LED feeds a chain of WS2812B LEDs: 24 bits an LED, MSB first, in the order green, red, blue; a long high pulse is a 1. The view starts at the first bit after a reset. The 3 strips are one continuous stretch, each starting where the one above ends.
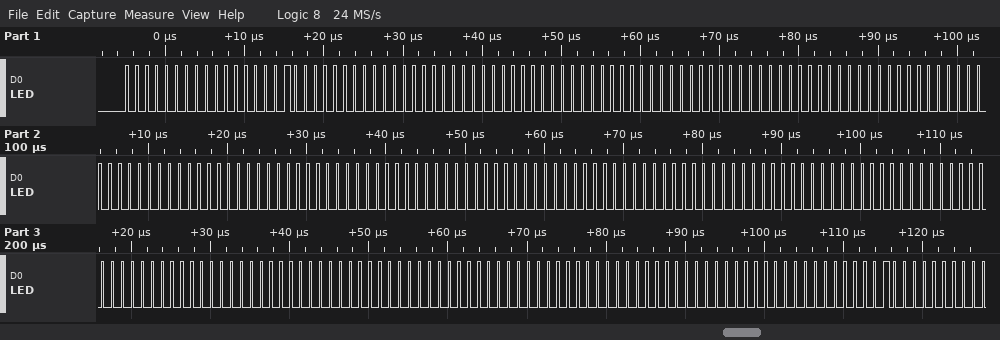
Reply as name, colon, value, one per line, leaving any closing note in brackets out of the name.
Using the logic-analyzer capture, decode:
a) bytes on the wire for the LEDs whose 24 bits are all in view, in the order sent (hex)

bytes on the wire for the LEDs whose 24 bits are all in view, in the order sent: 00 00 80 00 00 00 00 00 00 00 00 00 00 00 00 00 00 00 00 00 00 00 00 00 00 00 00 00 00 00 00 00 80
